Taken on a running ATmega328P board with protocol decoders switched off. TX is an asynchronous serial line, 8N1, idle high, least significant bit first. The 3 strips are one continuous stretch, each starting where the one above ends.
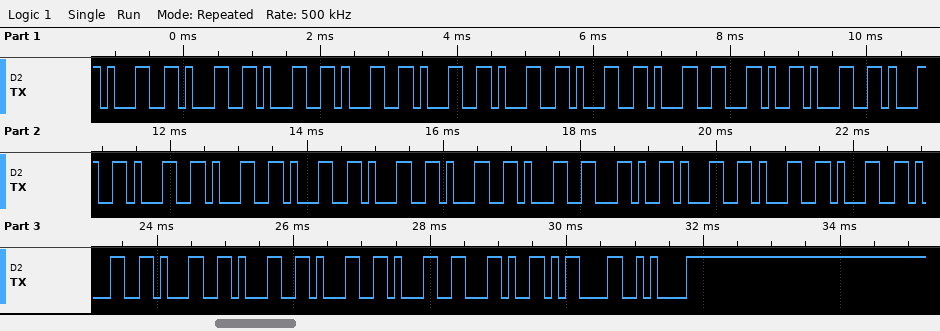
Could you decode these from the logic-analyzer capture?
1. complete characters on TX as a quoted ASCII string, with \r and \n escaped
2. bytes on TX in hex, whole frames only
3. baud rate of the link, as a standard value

"11111111,11111111,11111111,\r\n"
0x31 0x31 0x31 0x31 0x31 0x31 0x31 0x31 0x2C 0x31 0x31 0x31 0x31 0x31 0x31 0x31 0x31 0x2C 0x31 0x31 0x31 0x31 0x31 0x31 0x31 0x31 0x2C 0x0D 0x0A
9600 baud
